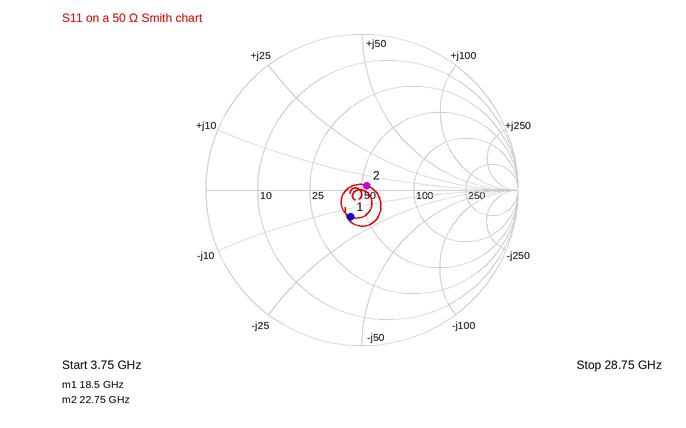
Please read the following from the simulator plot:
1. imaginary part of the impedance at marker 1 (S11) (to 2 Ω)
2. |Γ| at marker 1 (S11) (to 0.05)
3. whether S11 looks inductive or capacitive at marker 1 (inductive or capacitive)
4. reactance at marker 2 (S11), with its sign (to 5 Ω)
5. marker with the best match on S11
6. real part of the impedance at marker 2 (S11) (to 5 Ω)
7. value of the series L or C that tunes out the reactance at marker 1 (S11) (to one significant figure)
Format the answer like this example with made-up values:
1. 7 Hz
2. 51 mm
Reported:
1. -14 Ω
2. 0.20
3. capacitive
4. +5 Ω
5. marker 2
6. 55 Ω
7. 100 pH
